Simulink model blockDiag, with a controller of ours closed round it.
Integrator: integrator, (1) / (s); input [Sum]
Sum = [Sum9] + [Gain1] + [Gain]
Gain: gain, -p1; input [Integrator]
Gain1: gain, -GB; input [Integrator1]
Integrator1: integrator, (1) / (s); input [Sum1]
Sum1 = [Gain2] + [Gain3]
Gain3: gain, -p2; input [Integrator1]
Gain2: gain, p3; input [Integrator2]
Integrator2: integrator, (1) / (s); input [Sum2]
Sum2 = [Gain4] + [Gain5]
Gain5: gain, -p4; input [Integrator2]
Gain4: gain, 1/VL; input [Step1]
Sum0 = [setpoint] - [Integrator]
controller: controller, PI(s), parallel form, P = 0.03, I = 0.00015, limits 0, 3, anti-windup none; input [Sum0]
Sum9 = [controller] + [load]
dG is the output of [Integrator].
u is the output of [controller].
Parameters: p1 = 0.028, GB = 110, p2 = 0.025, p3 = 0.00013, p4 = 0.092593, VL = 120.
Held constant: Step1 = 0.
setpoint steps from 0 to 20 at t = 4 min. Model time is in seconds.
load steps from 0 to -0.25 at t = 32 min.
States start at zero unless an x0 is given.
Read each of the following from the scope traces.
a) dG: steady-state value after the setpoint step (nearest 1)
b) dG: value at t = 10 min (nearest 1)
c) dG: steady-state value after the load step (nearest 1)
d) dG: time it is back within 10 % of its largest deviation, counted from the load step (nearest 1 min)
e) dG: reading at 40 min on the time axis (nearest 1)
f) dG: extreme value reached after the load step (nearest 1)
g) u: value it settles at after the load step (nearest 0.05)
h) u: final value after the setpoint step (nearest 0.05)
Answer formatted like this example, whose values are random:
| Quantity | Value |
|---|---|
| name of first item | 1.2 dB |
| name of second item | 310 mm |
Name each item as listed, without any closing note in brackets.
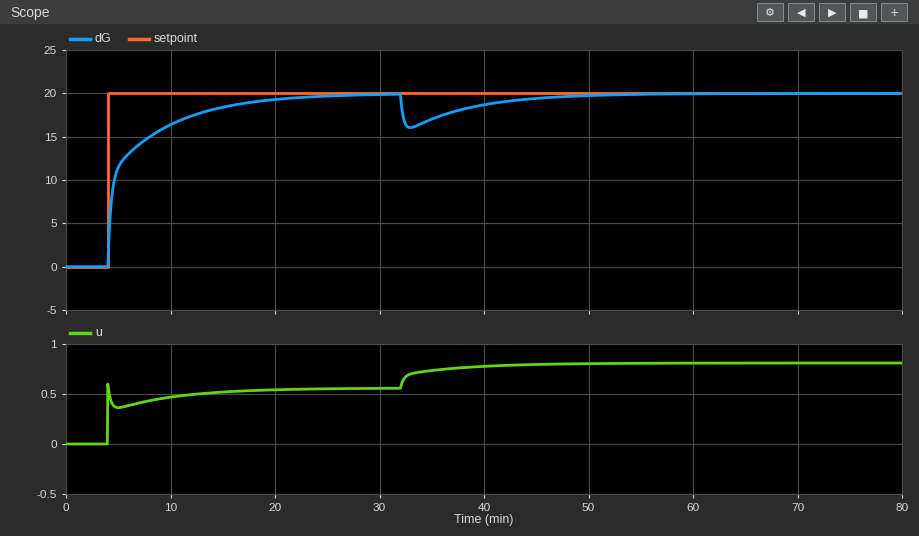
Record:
| Quantity | Value |
|---|---|
| dG: steady-state value after the setpoint step | 20 |
| dG: value at t = 10 min | 16 |
| dG: steady-state value after the load step | 20 |
| dG: time it is back within 10 % of its largest deviation, counted from the load step | 16 min |
| dG: reading at 40 min on the time axis | 19 |
| dG: extreme value reached after the load step | 16 |
| u: value it settles at after the load step | 0.80 |
| u: final value after the setpoint step | 0.55 |
